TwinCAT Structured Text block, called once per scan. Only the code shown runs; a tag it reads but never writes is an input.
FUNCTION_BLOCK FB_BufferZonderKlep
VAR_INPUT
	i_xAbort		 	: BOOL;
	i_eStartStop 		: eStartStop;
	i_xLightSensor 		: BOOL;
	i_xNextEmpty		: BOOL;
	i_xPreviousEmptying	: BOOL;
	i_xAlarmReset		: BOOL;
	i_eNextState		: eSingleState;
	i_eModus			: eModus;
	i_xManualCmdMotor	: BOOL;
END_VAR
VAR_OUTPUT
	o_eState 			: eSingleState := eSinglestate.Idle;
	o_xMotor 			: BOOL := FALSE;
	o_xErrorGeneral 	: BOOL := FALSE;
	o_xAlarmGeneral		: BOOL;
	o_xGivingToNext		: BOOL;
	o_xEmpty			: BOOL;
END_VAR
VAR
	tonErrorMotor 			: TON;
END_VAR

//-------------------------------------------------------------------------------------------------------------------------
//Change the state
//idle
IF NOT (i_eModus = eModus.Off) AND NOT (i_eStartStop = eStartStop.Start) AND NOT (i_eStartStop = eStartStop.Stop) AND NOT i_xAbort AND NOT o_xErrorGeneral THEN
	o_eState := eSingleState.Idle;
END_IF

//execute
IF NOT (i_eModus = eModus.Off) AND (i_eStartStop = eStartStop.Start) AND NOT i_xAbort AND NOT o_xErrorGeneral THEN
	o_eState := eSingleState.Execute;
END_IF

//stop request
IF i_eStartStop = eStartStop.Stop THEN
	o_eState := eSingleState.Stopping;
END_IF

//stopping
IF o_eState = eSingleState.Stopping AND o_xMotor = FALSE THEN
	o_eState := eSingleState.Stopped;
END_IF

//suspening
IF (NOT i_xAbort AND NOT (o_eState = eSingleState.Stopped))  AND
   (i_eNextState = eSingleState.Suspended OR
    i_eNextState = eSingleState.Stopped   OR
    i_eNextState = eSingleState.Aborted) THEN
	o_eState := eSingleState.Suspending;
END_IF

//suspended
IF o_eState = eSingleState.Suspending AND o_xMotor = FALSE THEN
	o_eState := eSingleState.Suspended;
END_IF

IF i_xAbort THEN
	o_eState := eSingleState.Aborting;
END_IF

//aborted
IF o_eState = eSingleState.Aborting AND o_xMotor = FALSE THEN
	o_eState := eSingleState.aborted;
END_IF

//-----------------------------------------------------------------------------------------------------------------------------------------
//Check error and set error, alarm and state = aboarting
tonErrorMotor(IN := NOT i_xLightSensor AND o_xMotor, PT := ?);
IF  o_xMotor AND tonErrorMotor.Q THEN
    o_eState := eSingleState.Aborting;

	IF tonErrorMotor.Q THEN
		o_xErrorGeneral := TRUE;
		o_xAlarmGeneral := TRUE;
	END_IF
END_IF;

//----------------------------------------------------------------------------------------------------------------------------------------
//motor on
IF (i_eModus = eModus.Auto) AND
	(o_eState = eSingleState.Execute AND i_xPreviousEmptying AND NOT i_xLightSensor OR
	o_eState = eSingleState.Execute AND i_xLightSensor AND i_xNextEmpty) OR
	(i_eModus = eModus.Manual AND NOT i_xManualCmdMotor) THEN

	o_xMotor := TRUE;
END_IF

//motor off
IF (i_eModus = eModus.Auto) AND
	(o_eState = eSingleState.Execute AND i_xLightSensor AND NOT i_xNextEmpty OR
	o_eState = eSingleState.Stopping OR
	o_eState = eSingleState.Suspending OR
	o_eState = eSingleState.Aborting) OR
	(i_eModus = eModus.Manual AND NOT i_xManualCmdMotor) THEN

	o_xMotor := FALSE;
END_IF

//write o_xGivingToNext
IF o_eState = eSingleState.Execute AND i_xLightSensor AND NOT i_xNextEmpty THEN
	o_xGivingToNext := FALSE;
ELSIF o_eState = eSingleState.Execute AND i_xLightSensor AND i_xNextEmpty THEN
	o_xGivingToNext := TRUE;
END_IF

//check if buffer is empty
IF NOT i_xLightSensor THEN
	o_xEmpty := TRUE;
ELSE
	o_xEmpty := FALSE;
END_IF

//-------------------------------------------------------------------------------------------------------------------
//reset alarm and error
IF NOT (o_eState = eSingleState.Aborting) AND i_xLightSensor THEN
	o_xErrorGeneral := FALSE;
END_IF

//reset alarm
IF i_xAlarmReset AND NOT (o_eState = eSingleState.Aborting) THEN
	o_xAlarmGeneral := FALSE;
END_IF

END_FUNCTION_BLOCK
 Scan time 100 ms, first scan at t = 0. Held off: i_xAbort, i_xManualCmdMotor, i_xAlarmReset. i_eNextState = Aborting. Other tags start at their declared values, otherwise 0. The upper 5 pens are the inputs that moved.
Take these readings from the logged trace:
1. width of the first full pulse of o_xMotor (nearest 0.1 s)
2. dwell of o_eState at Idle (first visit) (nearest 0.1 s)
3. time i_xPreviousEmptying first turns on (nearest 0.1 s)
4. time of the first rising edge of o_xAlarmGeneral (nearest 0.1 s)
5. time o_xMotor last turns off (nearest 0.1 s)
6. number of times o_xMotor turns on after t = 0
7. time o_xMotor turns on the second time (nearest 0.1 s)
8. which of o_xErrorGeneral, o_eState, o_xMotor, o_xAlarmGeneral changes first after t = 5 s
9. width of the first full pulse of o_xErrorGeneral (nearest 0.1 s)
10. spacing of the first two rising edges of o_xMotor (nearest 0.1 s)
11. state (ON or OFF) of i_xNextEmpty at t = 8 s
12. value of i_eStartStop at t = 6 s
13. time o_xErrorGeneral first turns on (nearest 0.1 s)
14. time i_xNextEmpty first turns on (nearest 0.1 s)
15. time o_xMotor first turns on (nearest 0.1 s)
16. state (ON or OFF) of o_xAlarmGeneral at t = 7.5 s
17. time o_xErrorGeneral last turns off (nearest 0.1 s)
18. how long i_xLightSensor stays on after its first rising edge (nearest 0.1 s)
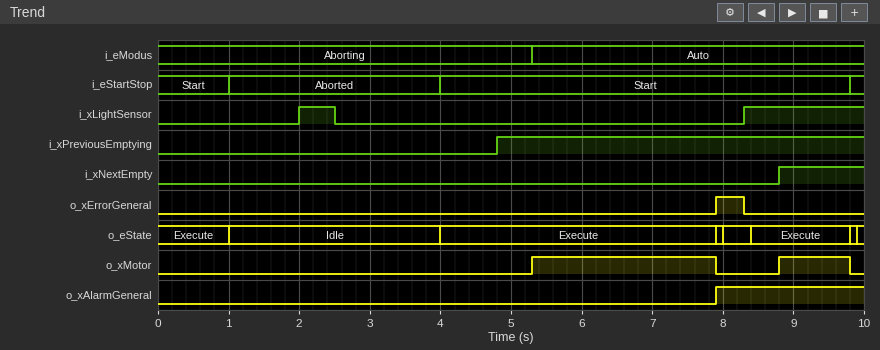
2.6 s
3.0 s
4.8 s
7.9 s
9.8 s
2
8.8 s
o_xMotor
0.4 s
3.5 s
OFF
Start
7.9 s
8.8 s
5.3 s
OFF
8.3 s
0.5 s
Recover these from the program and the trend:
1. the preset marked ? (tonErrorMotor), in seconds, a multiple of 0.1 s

2.5 s
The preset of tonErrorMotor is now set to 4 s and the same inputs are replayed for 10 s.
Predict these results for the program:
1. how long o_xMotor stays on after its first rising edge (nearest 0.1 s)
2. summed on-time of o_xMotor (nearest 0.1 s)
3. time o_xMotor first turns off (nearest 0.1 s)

3.0 s
4.0 s
8.3 s
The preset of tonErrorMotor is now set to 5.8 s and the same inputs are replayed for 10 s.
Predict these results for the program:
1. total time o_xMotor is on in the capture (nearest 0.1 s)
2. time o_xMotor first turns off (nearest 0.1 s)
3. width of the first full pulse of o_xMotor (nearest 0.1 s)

4.0 s
8.3 s
3.0 s
